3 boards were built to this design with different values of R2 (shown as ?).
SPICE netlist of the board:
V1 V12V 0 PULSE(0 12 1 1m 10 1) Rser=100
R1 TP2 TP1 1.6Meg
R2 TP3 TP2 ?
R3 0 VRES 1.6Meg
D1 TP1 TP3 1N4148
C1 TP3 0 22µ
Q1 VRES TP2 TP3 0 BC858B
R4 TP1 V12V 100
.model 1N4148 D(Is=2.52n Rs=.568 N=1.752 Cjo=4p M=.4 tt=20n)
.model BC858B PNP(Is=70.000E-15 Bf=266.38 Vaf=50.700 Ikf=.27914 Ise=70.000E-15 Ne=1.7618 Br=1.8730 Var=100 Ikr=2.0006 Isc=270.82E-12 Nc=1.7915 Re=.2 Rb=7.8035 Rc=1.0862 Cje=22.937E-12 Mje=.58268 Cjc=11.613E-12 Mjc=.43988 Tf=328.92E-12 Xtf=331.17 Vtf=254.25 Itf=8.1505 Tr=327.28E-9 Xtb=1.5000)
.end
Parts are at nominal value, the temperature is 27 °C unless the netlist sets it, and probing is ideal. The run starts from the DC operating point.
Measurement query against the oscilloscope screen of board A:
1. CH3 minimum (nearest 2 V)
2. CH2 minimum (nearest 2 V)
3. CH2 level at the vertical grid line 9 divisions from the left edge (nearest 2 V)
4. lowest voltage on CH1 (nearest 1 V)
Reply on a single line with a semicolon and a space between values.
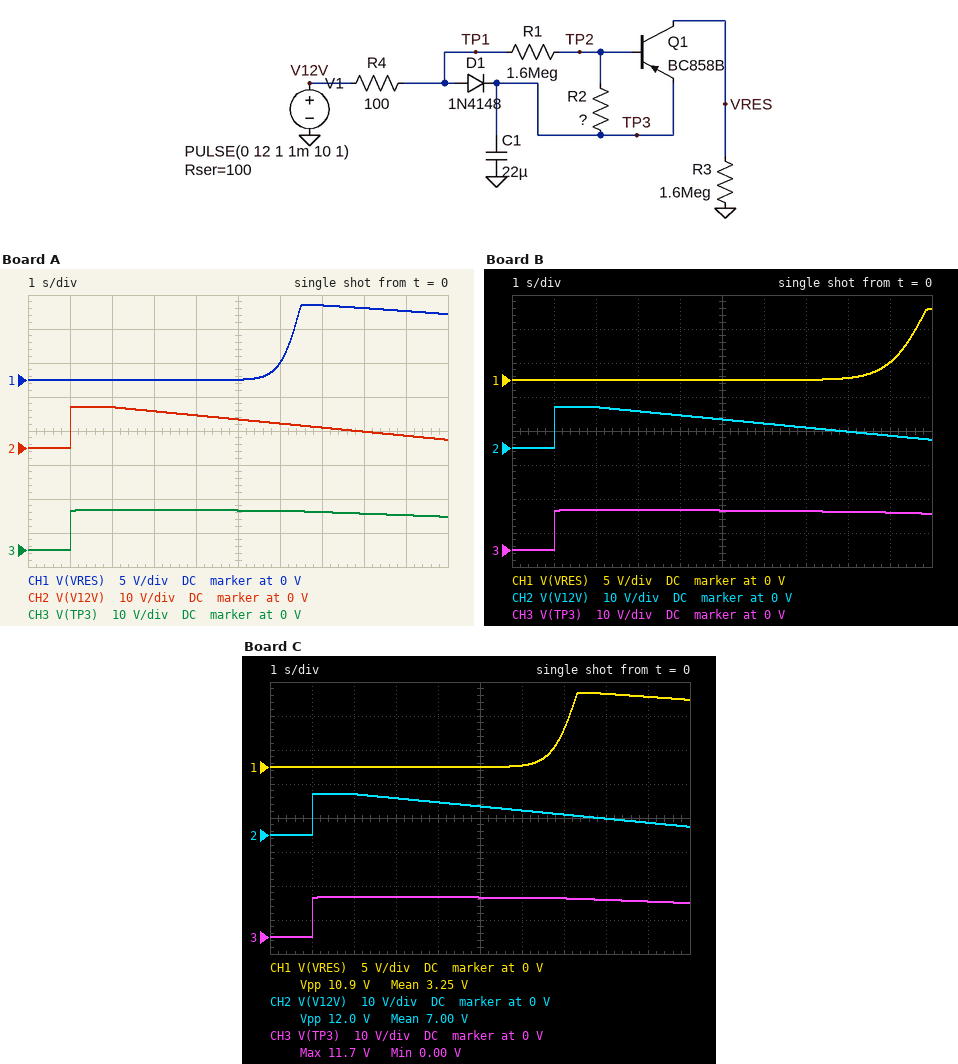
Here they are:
0 V; 0 V; 4 V; 0 V
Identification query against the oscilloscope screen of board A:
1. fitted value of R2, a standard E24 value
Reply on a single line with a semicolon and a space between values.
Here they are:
180 kΩ
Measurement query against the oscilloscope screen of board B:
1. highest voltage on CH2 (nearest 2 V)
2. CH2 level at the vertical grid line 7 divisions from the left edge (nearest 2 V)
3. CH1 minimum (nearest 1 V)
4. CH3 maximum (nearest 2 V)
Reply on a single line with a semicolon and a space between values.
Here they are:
12 V; 6 V; 0 V; 12 V
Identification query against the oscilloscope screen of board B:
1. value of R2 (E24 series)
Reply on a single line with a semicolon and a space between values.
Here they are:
100 kΩ
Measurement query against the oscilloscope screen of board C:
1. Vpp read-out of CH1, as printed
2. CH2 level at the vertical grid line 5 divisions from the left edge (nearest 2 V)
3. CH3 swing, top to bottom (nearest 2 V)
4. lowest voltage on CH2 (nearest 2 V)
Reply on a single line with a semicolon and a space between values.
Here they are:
10.9 V; 8 V; 12 V; 0 V
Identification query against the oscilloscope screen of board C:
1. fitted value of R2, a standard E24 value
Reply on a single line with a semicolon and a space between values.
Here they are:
150 kΩ
